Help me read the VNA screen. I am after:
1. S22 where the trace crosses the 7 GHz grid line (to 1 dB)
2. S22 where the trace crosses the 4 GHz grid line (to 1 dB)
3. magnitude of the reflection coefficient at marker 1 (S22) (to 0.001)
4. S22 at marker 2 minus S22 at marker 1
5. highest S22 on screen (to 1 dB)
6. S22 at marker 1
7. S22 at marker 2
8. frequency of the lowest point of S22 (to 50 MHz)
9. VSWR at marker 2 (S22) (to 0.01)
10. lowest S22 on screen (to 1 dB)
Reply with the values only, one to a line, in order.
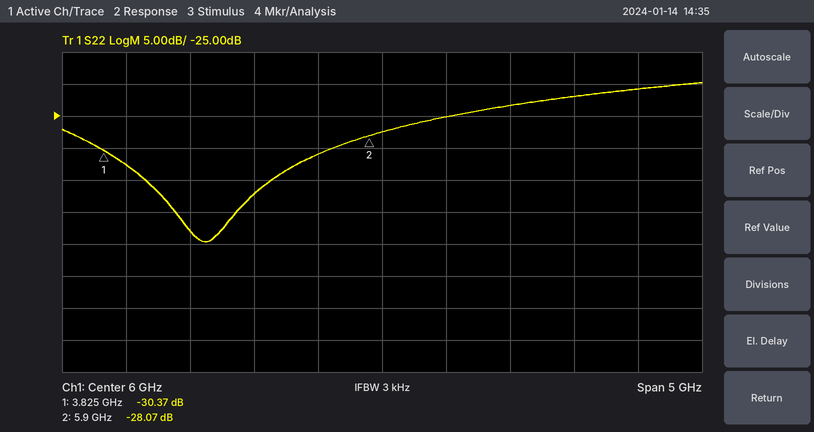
-23 dB
-33 dB
0.030
2.30 dB
-20 dB
-30.37 dB
-28.07 dB
4.60 GHz
1.08
-45 dB
